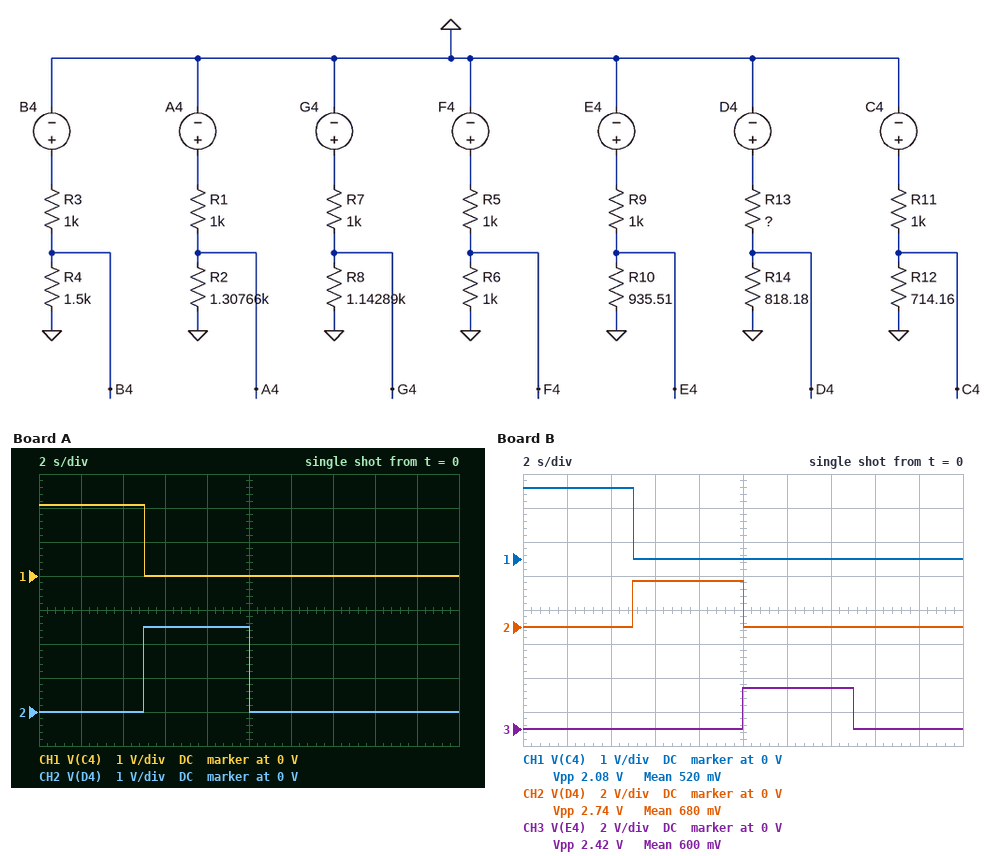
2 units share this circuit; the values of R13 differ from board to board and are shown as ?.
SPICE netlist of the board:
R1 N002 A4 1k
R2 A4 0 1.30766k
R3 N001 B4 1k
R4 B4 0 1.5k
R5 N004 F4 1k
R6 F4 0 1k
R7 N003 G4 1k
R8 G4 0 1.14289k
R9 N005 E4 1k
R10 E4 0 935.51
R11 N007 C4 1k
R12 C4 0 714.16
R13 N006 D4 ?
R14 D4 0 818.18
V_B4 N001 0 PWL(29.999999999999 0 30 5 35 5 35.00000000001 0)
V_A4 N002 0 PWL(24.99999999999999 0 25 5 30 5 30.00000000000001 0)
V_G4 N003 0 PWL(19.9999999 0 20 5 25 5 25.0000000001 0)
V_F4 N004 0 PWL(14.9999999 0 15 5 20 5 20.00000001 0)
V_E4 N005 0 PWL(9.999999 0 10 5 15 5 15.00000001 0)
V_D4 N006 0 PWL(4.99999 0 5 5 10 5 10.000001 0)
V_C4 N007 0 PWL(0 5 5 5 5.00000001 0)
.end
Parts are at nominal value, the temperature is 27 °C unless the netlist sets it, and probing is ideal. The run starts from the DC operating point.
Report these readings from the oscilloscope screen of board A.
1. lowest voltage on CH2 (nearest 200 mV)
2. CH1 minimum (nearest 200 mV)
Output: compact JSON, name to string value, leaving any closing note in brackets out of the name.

{"lowest voltage on CH2": "0 V", "CH1 minimum": "0 V"}
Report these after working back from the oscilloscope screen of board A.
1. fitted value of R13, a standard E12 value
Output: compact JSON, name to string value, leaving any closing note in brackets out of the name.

{"fitted value of R13, a standard E12 value": "820 Ω"}
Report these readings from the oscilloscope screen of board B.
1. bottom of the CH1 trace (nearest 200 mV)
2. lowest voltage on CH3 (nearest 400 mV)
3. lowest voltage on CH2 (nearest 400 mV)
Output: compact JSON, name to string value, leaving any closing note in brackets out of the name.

{"bottom of the CH1 trace": "0 V", "lowest voltage on CH3": "0 V", "lowest voltage on CH2": "0 V"}
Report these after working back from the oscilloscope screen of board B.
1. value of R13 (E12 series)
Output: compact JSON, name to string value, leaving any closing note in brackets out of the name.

{"value of R13": "680 Ω"}
